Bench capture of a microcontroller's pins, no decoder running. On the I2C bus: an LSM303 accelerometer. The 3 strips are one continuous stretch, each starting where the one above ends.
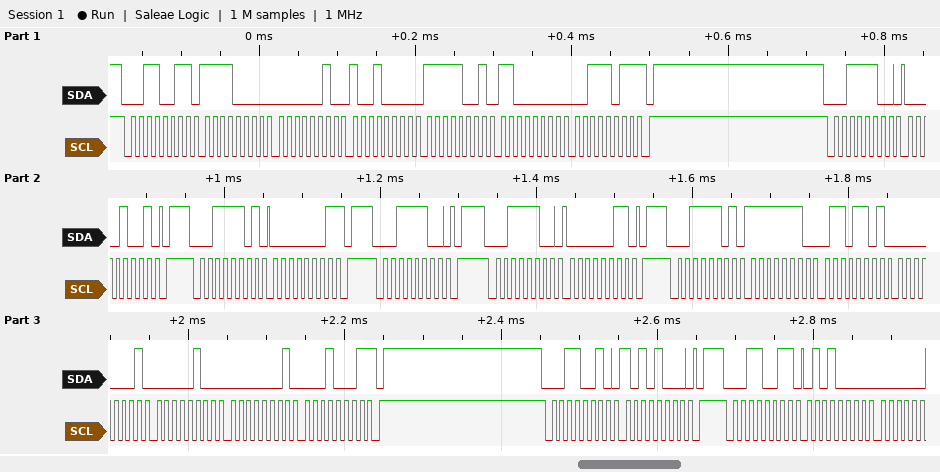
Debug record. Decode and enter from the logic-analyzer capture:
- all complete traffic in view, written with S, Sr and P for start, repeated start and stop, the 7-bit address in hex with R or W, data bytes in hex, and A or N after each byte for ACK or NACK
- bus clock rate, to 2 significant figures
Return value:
S 19R A F0 A 02 A 90 A F9 A C0 A 3B N P S 1EW A 09 A P S 1ER A 01 N P S 1EW A P S 1EW A 03 A P S 1ER A FE A 6D A 01 A 04 A 01 A 11 N P S 19W A A8 A P S 19R A 50 A
100 kHz
